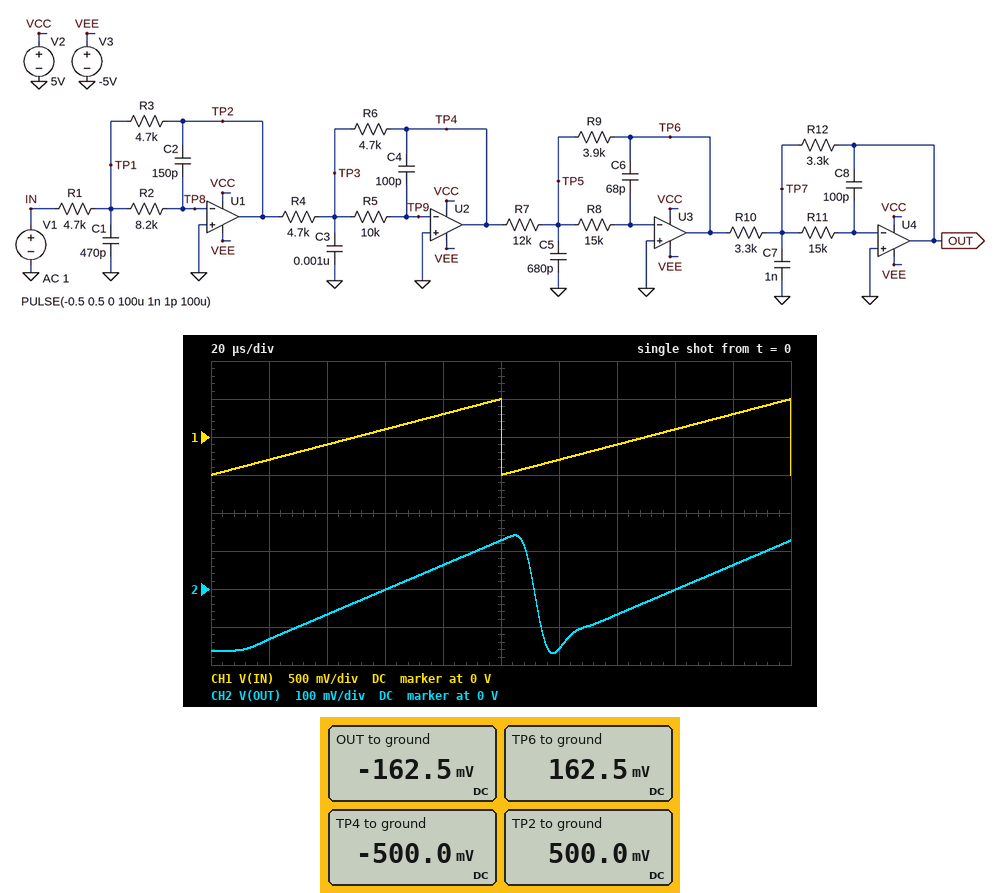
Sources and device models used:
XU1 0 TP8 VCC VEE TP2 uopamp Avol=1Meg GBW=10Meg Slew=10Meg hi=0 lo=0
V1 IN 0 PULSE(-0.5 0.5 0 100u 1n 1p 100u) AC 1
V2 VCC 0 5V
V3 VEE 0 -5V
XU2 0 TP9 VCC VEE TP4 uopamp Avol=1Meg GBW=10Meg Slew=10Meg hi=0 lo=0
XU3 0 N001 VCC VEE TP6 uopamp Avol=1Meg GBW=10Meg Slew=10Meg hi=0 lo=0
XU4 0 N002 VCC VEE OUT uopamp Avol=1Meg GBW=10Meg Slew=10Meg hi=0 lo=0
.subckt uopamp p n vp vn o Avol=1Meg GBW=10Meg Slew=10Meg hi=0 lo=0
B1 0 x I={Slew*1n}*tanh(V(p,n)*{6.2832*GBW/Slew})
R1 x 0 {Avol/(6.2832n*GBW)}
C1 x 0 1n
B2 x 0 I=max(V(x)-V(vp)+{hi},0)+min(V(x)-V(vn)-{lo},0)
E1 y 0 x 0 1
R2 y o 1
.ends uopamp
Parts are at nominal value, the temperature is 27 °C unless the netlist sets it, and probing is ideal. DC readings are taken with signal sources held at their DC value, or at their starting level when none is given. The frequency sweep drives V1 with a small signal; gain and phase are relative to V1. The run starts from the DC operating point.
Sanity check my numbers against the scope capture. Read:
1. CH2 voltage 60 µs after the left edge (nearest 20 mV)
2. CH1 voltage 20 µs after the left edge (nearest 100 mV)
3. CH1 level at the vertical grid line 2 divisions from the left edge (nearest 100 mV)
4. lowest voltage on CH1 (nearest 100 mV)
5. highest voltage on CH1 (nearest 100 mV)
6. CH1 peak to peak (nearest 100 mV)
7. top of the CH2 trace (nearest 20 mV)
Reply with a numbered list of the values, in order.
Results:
1. 0 V
2. -300 mV
3. -100 mV
4. -500 mV
5. 500 mV
6. 1.0 V
7. 140 mV
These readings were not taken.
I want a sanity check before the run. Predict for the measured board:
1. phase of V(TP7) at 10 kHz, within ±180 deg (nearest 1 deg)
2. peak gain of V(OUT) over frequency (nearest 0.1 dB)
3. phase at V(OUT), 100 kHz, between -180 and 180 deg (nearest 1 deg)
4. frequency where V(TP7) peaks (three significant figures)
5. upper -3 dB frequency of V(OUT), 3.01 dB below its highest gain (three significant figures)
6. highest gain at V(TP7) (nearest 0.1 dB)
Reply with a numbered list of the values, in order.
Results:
1. -129 deg
2. -9.8 dB
3. -64 deg
4. 53.1 kHz
5. 57.9 kHz
6. -17.8 dB
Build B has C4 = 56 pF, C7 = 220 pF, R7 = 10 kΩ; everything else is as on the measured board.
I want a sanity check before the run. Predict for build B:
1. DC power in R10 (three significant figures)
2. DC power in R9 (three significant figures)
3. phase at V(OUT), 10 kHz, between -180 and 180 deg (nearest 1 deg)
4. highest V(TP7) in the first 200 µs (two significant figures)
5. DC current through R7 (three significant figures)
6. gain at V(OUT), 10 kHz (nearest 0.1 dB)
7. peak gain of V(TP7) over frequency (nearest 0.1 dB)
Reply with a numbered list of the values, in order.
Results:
1. 11.5 µW
2. 9.75 µW
3. -35 deg
4. 84 mV
5. 50.0 µA
6. -8.3 dB
7. -16.2 dB
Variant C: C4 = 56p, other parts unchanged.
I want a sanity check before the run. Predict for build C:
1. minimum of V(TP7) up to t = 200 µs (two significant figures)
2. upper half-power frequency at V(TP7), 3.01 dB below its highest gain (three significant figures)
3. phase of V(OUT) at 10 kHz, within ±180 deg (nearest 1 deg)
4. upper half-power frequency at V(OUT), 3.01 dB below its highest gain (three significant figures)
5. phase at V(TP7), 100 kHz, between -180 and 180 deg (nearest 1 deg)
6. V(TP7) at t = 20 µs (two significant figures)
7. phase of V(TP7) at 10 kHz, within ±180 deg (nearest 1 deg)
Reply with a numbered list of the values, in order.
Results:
1. -19 mV
2. 88.8 kHz
3. -35 deg
4. 69.0 kHz
5. -128 deg
6. -5.0 mV
7. -125 deg
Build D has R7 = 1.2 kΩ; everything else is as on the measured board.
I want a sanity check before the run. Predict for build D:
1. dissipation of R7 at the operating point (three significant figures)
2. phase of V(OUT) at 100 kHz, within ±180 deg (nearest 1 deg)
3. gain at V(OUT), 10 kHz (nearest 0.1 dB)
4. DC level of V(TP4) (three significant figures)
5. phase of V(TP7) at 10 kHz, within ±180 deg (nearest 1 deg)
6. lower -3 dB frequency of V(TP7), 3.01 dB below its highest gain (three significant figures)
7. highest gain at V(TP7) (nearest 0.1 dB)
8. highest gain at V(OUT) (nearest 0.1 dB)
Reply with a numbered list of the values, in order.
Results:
1. 208 µW
2. -61 deg
3. 9.9 dB
4. -500 mV
5. -139 deg
6. 19.2 kHz
7. -2.6 dB
8. 10.2 dB
